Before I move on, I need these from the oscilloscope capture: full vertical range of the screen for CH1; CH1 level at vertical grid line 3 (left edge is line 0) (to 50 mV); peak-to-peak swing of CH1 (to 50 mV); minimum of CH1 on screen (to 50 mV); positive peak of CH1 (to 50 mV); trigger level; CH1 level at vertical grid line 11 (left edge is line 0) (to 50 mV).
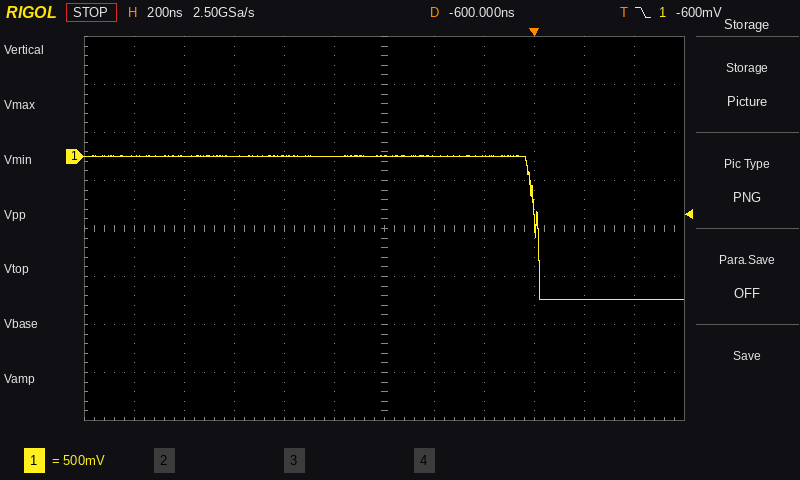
4 V
0 mV
1.50 V
-1.50 V
0 mV
-600 mV
-1.50 V
